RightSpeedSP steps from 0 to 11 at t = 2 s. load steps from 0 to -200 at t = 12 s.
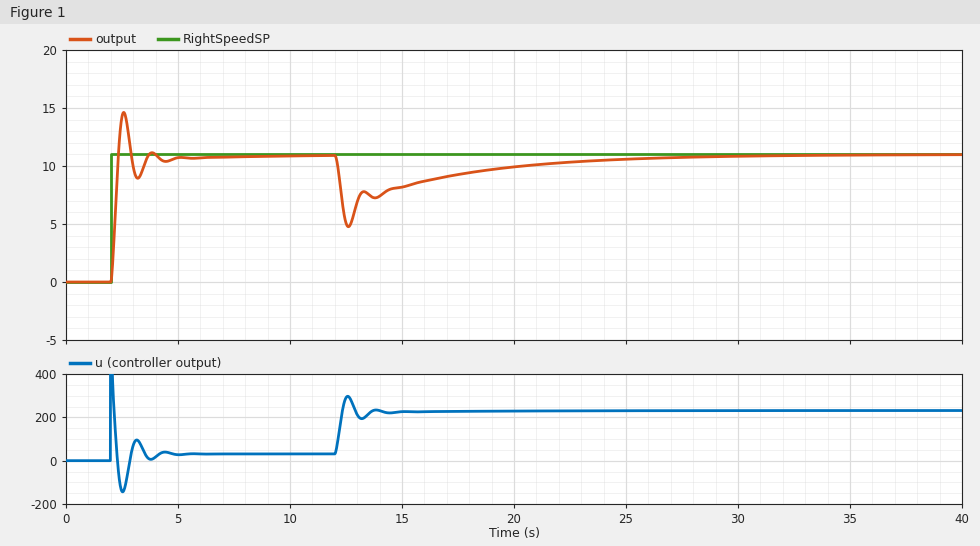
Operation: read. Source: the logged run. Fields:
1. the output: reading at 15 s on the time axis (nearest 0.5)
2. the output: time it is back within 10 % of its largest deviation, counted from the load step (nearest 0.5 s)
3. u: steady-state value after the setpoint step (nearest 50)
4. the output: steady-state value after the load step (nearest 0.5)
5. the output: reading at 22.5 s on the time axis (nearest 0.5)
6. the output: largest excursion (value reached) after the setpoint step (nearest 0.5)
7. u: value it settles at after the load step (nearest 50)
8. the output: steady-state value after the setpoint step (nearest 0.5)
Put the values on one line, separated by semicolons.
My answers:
8.0; 11.0 s; 50; 11.0; 10.5; 14.5; 250; 11.0
